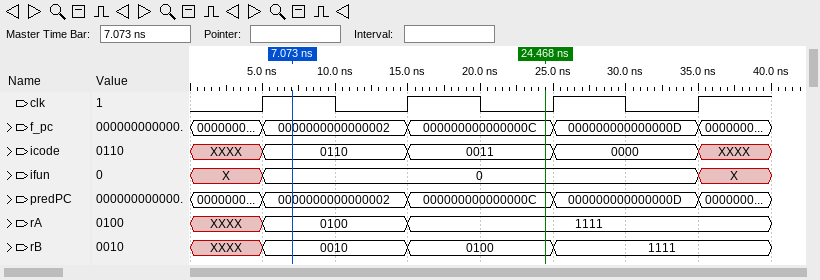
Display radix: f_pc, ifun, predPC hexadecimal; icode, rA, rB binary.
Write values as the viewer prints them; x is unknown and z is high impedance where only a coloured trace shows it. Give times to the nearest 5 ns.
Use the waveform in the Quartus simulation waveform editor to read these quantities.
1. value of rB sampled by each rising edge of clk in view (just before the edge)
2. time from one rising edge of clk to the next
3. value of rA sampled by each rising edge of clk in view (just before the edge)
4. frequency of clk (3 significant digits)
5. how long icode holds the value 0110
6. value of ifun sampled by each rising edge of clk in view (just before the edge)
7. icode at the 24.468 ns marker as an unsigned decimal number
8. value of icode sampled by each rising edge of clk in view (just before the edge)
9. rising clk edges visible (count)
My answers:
XXXX, 0010, 0100, 1111
10 ns
XXXX, 0100, 1111, 1111
100 MHz
10 ns
X, 0, 0, 0
3
XXXX, 0110, 0011, 0000
4
